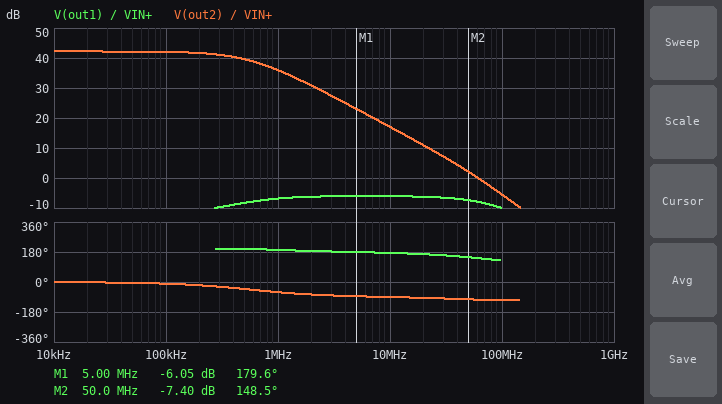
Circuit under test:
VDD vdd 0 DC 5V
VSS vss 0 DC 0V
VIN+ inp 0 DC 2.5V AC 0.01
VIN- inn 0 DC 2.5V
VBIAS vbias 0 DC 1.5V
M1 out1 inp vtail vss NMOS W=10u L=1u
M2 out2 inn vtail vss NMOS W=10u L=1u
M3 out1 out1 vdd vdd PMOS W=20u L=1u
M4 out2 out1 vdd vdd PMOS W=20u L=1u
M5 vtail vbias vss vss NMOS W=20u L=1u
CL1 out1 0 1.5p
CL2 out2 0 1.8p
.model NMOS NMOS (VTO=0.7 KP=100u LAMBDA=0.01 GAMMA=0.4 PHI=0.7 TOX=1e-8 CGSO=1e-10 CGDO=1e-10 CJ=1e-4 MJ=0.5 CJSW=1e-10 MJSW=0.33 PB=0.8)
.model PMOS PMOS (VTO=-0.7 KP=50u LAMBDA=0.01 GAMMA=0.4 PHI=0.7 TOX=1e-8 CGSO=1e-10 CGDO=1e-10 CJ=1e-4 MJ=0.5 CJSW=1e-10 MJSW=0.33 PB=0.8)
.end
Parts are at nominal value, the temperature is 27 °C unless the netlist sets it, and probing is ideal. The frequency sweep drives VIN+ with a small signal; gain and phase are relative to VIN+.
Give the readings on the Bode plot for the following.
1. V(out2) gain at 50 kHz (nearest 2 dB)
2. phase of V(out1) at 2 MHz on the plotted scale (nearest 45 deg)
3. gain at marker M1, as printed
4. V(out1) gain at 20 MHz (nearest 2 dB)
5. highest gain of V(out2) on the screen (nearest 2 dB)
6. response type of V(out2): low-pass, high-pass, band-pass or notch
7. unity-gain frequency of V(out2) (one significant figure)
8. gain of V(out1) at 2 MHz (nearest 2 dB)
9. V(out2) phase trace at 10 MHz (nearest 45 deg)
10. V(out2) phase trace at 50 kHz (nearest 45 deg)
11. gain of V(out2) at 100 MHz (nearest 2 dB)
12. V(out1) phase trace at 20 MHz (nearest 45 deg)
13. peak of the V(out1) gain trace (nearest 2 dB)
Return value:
42 dB
180 deg
-6.05 dB
-6 dB
42 dB
low-pass
60 MHz
-6 dB
-90 deg
0 deg
-6 dB
180 deg
-6 dB
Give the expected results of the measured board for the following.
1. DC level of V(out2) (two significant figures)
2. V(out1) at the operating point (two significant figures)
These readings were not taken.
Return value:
3.5 V
3.5 V
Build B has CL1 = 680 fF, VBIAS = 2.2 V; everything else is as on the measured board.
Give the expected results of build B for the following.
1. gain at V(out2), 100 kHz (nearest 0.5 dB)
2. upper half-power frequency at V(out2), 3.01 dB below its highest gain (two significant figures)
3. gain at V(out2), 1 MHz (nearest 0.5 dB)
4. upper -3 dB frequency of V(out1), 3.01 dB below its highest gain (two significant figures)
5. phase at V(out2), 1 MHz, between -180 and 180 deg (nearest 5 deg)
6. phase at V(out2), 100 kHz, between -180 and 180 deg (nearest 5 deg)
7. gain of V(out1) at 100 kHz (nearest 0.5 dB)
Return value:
39.0 dB
1.2 MHz
36.5 dB
240 MHz
-40 deg
-5 deg
-5.0 dB
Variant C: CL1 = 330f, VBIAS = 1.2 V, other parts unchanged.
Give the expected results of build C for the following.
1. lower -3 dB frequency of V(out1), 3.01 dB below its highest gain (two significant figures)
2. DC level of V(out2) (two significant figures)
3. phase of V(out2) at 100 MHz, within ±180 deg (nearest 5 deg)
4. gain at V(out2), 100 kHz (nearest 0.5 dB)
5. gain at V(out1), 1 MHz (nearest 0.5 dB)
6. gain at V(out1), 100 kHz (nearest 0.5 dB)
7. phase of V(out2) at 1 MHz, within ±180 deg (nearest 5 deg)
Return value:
150 kHz
3.8 V
-105 deg
45.5 dB
-6.0 dB
-10.0 dB
-80 deg
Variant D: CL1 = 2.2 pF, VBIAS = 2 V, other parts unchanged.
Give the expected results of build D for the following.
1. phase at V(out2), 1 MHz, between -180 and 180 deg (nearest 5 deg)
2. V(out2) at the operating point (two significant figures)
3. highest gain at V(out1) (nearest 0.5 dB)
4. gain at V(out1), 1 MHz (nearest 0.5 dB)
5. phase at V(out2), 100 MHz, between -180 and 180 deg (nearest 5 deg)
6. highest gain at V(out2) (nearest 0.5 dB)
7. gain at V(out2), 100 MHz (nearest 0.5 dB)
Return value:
-45 deg
3.2 V
-3.5 dB
-4.5 dB
-120 deg
39.5 dB
-4.0 dB
